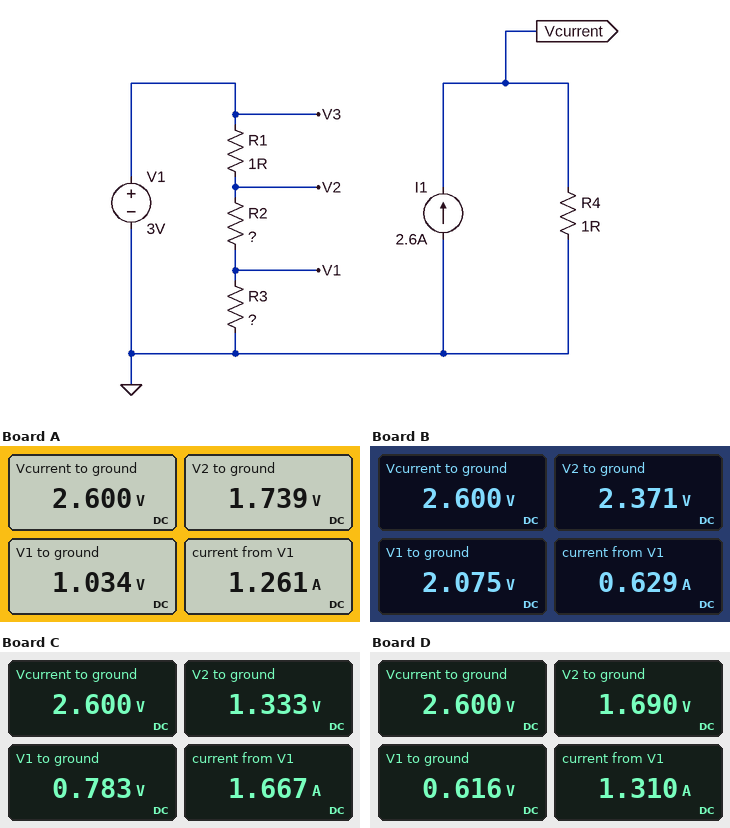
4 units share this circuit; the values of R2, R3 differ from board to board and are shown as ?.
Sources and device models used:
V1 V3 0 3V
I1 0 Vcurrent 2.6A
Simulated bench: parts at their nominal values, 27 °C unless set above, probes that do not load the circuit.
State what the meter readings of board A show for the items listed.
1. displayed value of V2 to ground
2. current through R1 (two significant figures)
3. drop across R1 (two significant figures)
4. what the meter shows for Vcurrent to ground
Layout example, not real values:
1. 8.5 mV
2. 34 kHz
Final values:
1. 1.739 V
2. 1.3 A
3. 1.3 V
4. 2.600 V
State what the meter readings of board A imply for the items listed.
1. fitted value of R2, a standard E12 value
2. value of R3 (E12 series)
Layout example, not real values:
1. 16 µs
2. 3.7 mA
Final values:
1. 0.56 Ω
2. 0.82 Ω
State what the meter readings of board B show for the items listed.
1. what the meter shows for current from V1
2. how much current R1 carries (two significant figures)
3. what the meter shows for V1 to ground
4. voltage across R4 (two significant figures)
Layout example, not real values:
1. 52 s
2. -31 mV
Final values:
1. 0.629 A
2. 630 mA
3. 2.075 V
4. 2.6 V
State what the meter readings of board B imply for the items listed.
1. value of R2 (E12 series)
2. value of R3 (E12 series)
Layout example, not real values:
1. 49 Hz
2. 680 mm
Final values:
1. 0.47 Ω
2. 3.3 Ω
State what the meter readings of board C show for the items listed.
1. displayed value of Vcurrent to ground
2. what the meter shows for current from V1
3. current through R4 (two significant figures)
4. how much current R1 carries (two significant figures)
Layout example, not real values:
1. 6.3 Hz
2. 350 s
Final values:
1. 2.600 V
2. 1.667 A
3. 2.6 A
4. 1.7 A
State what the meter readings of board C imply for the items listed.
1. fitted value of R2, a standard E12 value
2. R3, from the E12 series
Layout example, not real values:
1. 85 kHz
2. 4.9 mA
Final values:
1. 0.33 Ω
2. 0.47 Ω
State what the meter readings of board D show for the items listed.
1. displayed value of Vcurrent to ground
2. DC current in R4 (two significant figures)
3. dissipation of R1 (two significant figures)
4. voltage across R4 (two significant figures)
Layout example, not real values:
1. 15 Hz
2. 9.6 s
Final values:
1. 2.600 V
2. 2.6 A
3. 1.7 W
4. 2.6 V
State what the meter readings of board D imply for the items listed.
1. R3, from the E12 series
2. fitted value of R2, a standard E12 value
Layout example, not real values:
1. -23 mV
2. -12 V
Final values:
1. 0.47 Ω
2. 0.82 Ω
